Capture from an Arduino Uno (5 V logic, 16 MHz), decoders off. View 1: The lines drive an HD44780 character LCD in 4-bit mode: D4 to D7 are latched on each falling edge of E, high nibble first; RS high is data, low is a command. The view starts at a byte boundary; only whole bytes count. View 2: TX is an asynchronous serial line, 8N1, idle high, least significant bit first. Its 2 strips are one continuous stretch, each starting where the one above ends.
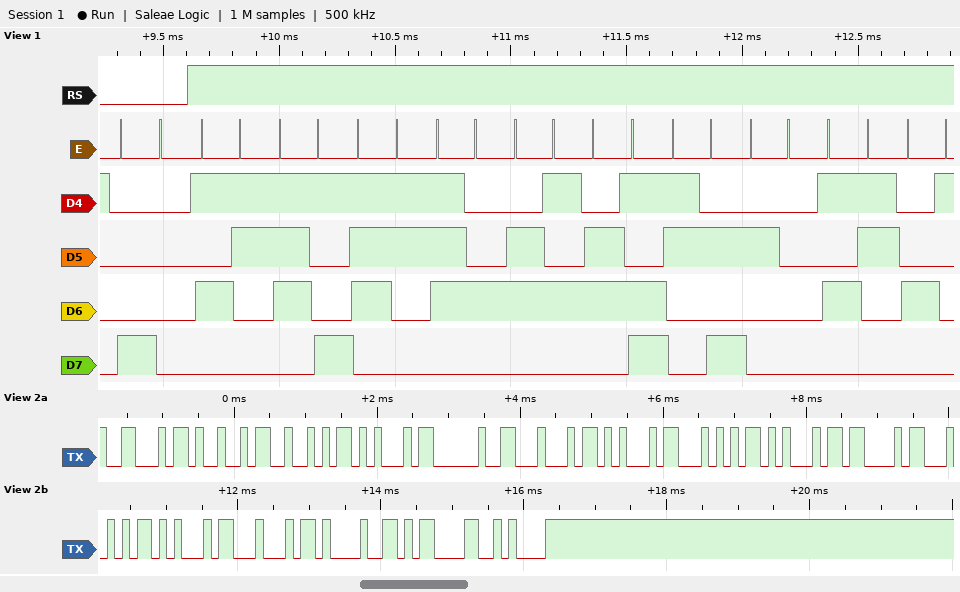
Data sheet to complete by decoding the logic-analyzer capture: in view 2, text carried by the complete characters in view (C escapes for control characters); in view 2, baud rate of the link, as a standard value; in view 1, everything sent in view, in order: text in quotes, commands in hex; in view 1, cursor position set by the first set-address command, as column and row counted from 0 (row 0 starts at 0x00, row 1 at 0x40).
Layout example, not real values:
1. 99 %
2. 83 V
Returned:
1. "FIRE DETECTED!\r\n"
2. 9600 baud
3. 0x80 "System: SA"
4. column 0, row 0
